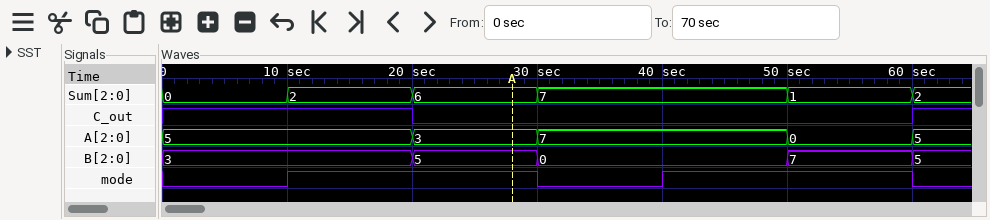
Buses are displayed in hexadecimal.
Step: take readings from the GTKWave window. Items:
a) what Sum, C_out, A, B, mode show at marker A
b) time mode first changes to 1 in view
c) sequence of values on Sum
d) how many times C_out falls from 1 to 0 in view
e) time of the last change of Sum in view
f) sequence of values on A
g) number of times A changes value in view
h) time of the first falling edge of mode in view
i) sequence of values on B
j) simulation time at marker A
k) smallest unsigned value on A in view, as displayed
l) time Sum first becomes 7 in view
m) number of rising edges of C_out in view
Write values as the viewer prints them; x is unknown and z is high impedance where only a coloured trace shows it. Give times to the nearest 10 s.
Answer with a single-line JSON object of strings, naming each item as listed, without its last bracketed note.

{"what Sum, C_out, A, B, mode show at marker A": "Sum=6, C_out=0, A=3, B=5, mode=1", "time mode first changes to 1 in view": "10 s", "sequence of values on Sum": "0, 2, 6, 7, 1, 2", "how many times C_out falls from 1 to 0 in view": "1", "time of the last change of Sum in view": "60 s", "sequence of values on A": "5, 3, 7, 0, 5", "number of times A changes value in view": "4", "time of the first falling edge of mode in view": "30 s", "sequence of values on B": "3, 5, 0, 7, 5", "simulation time at marker A": "30 s", "smallest unsigned value on A in view, as displayed": "0", "time Sum first becomes 7 in view": "30 s", "number of rising edges of C_out in view": "1"}
